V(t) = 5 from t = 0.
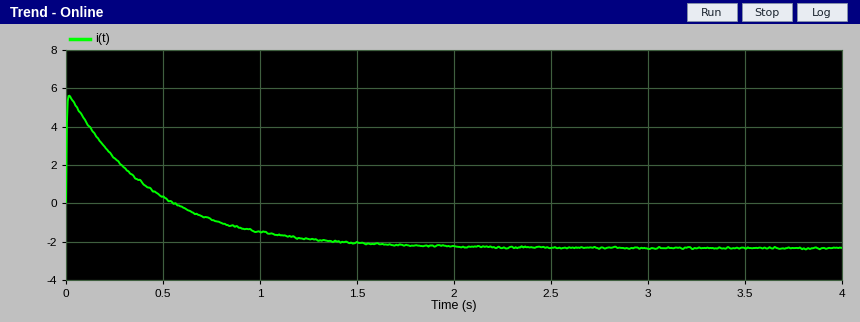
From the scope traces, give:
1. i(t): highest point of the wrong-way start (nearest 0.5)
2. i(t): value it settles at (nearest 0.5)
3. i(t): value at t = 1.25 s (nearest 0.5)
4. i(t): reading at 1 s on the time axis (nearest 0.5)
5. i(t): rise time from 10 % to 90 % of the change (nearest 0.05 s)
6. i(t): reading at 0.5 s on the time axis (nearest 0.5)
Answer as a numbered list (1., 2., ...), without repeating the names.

1. 5.5
2. -2.5
3. -2.0
4. -1.5
5. 0.95 s
6. 0.5
